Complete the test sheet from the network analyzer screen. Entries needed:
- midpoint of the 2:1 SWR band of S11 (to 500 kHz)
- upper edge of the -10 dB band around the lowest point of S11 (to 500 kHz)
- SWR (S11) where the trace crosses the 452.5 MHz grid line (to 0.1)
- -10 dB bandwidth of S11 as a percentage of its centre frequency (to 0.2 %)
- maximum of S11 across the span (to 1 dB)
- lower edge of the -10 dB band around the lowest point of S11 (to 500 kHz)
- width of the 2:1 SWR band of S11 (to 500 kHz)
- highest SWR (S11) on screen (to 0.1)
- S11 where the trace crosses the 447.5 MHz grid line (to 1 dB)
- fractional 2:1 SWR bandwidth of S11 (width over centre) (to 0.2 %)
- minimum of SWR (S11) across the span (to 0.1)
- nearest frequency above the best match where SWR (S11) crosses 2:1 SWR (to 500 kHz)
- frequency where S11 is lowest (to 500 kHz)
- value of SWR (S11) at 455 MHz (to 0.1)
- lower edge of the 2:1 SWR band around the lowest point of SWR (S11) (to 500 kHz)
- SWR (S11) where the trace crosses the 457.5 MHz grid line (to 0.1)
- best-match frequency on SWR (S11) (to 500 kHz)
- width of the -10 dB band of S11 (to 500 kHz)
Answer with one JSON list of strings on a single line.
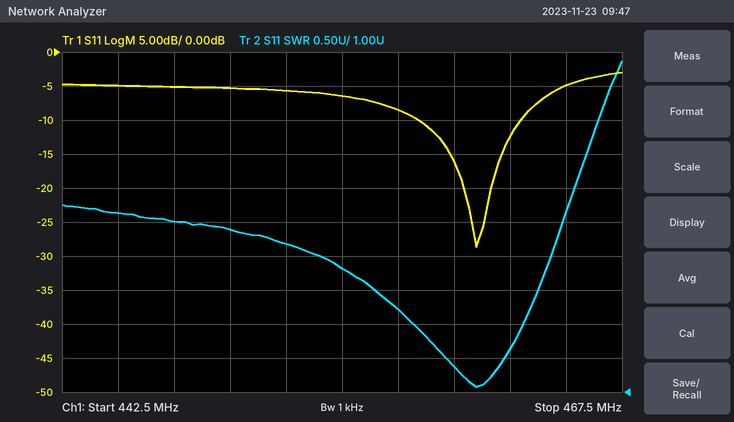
["460.5 MHz", "463.0 MHz", "3.2", "1.0 %", "-3 dB", "458.5 MHz", "5.0 MHz", "5.9", "-5 dB", "1.0 %", "1.1", "463.0 MHz", "461.0 MHz", "2.8", "458.0 MHz", "2.2", "461.0 MHz", "4.5 MHz"]
